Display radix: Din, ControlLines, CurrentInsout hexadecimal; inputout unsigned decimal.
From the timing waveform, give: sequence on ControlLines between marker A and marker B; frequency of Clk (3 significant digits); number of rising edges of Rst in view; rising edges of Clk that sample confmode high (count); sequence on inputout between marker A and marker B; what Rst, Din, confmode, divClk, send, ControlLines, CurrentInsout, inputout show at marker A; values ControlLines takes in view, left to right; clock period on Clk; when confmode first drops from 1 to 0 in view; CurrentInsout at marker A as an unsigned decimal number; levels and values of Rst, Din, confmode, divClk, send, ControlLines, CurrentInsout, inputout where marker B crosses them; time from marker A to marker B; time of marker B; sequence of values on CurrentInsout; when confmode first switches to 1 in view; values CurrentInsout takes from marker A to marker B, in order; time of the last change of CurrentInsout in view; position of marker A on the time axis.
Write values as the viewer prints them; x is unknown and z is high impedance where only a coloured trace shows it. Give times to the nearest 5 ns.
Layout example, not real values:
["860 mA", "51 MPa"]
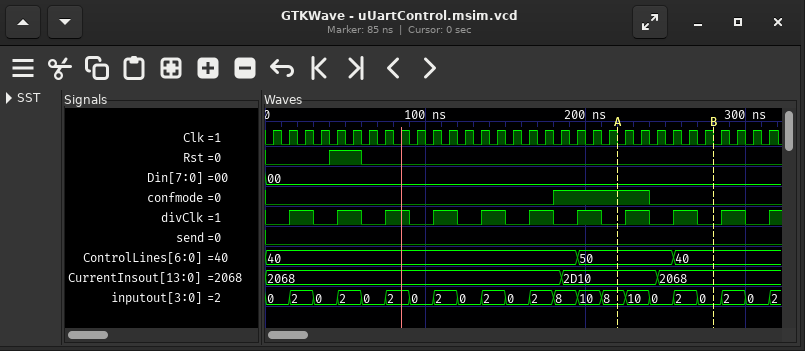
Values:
["50, 40", "100 MHz", "1", "6", "8, 10, 0, 2, 0", "Rst=0, Din=00, confmode=1, divClk=0, send=0, ControlLines=50, CurrentInsout=2D10, inputout=8", "40, 50, 40", "10 ns", "240 ns", "11536", "Rst=0, Din=00, confmode=0, divClk=0, send=0, ControlLines=40, CurrentInsout=2068, inputout=0", "60 ns", "280 ns", "2068, 2D10, 2068", "180 ns", "2D10, 2068", "245 ns", "220 ns"]
